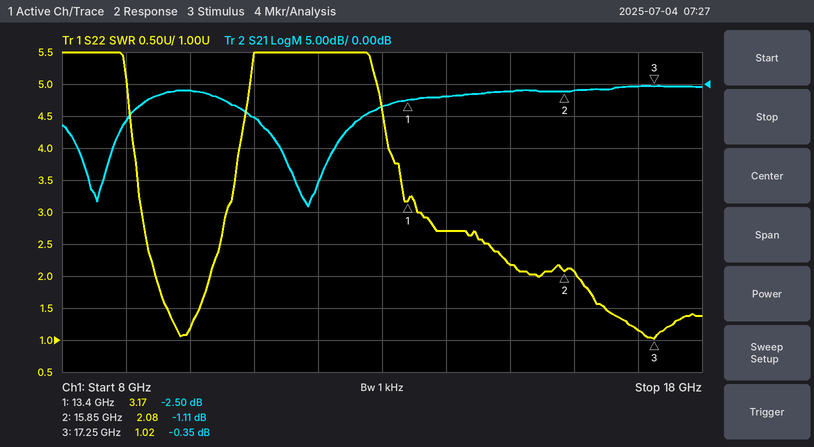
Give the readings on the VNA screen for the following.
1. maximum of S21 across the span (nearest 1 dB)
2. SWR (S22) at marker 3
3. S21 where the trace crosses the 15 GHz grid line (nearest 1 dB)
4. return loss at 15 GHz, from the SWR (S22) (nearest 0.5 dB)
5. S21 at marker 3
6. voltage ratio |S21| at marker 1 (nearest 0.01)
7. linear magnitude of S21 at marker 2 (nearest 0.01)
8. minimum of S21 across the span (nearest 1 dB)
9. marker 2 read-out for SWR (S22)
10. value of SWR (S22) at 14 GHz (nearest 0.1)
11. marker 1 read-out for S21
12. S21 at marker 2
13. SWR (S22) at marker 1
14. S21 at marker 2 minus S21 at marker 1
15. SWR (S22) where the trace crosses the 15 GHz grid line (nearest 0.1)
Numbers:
0 dB
1.02
-1 dB
8.5 dB
-0.35 dB
0.75
0.88
-19 dB
2.08
2.7
-2.50 dB
-1.11 dB
3.17
1.39 dB
2.2
